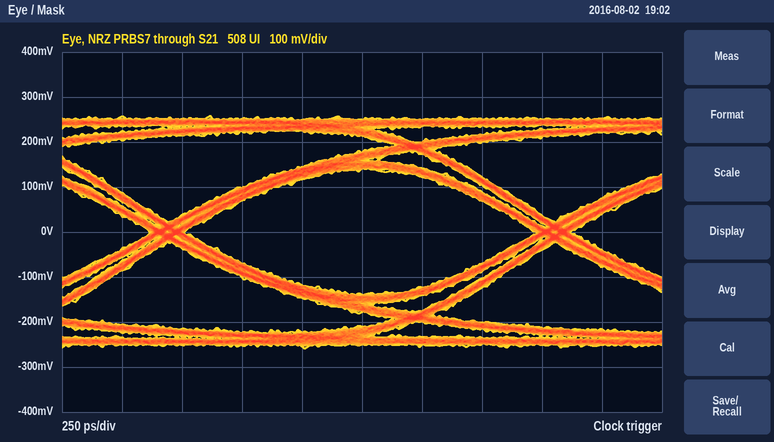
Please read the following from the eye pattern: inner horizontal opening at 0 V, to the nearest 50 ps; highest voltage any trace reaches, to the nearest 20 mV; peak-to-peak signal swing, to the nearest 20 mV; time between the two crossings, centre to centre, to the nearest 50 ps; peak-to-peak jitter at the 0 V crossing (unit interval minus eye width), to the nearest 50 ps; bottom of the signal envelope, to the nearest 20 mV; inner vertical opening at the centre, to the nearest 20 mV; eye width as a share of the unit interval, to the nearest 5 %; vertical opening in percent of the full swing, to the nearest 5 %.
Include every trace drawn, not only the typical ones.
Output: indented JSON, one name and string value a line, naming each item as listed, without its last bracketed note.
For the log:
{
  "inner horizontal opening at 0 V, to the nearest 50 ps": "1.45 ns",
  "highest voltage any trace reaches, to the nearest 20 mV": "260 mV",
  "peak-to-peak signal swing, to the nearest 20 mV": "520 mV",
  "time between the two crossings, centre to centre, to the nearest 50 ps": "1.60 ns",
  "peak-to-peak jitter at the 0 V crossing (unit interval minus eye width), to the nearest 50 ps": "150 ps",
  "bottom of the signal envelope, to the nearest 20 mV": "-260 mV",
  "inner vertical opening at the centre, to the nearest 20 mV": "280 mV",
  "eye width as a share of the unit interval, to the nearest 5 %": "90 %",
  "vertical opening in percent of the full swing, to the nearest 5 %": "55 %"
}
